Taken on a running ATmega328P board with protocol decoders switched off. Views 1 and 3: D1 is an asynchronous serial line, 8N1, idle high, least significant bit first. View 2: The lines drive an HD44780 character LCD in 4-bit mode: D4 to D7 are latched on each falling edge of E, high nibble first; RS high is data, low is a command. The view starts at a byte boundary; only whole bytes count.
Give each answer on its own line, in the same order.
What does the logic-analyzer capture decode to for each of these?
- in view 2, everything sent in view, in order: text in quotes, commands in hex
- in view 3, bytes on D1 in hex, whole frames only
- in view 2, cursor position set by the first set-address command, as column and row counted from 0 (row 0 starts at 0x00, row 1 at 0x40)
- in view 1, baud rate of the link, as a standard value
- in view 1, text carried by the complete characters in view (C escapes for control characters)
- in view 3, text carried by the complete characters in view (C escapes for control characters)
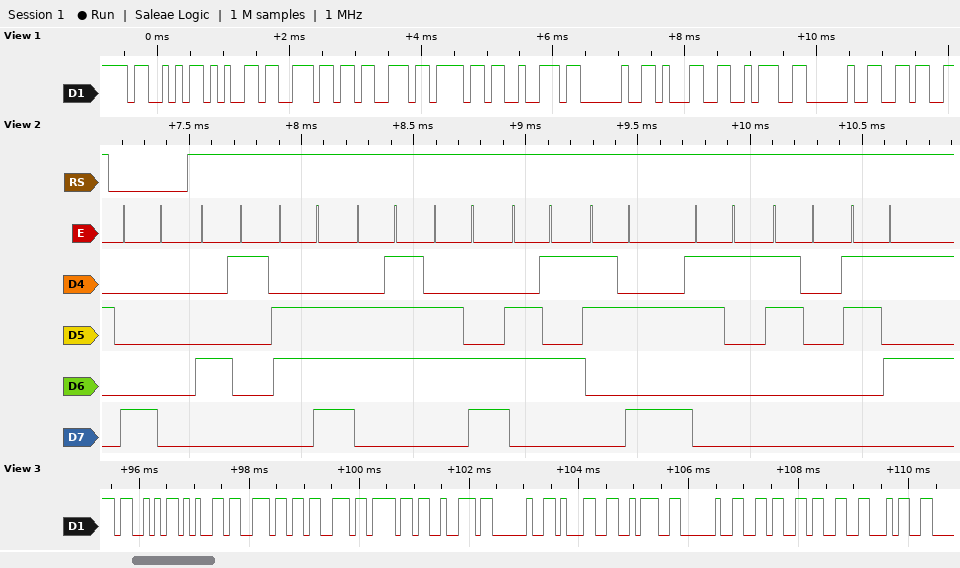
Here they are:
0x80 "Angle:105"
53 65 6E 73 6F 72 20 31 3A 20 36 33 34
column 0, row 0
9600 baud
"Sensor 1: 6"
"Sensor 1: 634"
